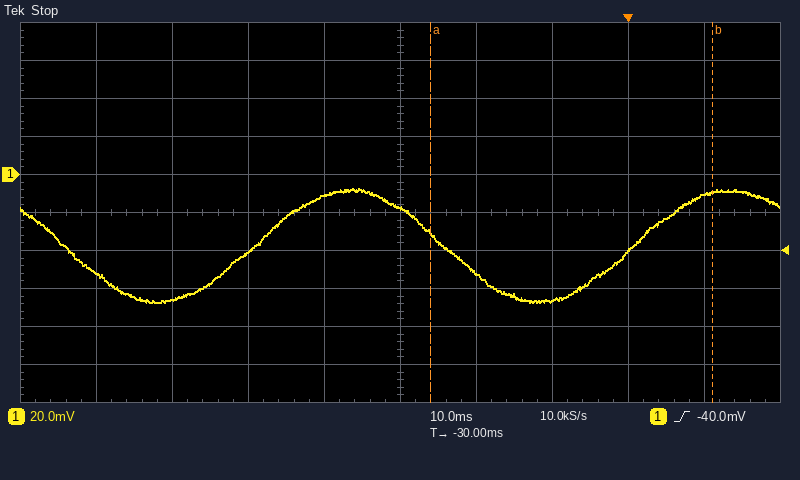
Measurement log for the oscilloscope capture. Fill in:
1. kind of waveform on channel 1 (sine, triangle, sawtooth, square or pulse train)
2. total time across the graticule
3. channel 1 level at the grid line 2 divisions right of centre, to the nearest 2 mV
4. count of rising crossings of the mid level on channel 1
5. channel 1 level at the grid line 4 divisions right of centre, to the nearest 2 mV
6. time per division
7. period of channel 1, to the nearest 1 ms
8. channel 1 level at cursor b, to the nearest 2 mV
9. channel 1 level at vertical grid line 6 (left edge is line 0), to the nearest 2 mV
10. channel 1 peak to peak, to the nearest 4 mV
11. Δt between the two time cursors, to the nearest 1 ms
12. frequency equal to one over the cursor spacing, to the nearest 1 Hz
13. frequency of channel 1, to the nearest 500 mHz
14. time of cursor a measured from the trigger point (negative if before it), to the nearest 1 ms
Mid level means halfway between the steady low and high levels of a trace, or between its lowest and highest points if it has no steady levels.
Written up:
sine
100 ms
-66 mV
2
-10 mV
10 ms
50 ms
-10 mV
-52 mV
60 mV
37 ms
27 Hz
20.0 Hz
-26 ms
